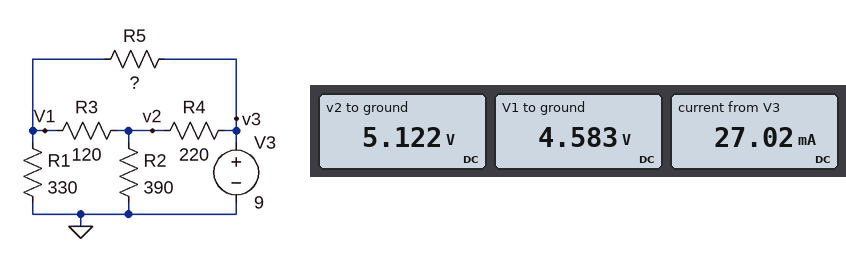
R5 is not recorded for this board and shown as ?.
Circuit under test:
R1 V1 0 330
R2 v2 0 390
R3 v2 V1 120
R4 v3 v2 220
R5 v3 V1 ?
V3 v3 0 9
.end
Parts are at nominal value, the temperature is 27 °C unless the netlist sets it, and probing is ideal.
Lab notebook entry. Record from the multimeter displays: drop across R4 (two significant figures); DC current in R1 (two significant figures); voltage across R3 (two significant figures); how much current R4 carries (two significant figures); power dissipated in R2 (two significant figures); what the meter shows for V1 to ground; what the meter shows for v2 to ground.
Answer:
3.9 V
14 mA
540 mV
18 mA
67 mW
4.583 V
5.122 V
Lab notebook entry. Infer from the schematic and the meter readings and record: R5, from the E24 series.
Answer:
470 Ω
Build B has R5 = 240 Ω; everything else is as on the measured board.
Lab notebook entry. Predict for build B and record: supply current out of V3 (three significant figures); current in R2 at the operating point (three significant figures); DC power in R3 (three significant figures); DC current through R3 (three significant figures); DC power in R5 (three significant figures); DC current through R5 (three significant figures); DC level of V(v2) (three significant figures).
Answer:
30.6 mA
14.3 mA
222 µW
1.36 mA
54.0 mW
15.0 mA
5.56 V
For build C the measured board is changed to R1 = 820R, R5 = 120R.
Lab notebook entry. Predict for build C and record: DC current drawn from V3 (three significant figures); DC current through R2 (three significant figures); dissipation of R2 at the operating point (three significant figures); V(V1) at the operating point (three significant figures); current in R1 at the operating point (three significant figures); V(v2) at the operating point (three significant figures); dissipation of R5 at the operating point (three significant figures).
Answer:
25.7 mA
16.8 mA
110 mW
7.25 V
8.84 mA
6.56 V
25.5 mW
